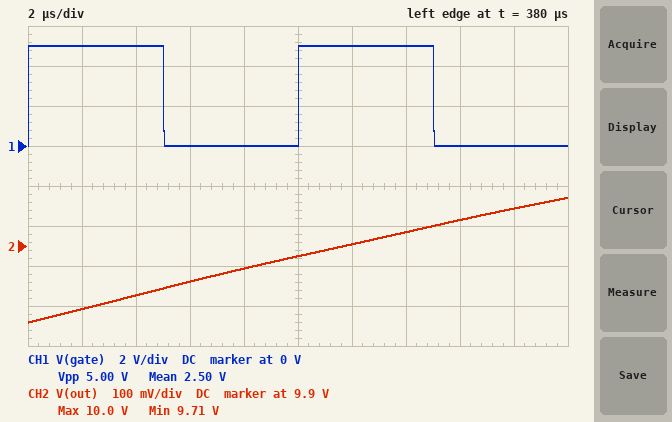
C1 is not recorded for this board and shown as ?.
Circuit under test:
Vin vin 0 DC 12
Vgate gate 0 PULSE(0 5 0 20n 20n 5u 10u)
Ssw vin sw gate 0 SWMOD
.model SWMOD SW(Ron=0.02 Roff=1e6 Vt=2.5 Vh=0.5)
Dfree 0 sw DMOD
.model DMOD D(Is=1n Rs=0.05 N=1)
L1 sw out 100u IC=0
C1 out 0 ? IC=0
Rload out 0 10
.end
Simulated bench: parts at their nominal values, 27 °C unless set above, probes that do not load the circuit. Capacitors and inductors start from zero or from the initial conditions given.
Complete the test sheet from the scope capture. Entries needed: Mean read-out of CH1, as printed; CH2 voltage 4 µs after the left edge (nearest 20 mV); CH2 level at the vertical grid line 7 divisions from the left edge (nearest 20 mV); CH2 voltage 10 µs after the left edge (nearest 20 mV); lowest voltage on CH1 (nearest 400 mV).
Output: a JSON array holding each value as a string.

["2.50 V", "9.78 V", "9.94 V", "9.88 V", "0 V"]
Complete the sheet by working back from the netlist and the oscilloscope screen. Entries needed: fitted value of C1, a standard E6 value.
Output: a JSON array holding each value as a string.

["220 µF"]
